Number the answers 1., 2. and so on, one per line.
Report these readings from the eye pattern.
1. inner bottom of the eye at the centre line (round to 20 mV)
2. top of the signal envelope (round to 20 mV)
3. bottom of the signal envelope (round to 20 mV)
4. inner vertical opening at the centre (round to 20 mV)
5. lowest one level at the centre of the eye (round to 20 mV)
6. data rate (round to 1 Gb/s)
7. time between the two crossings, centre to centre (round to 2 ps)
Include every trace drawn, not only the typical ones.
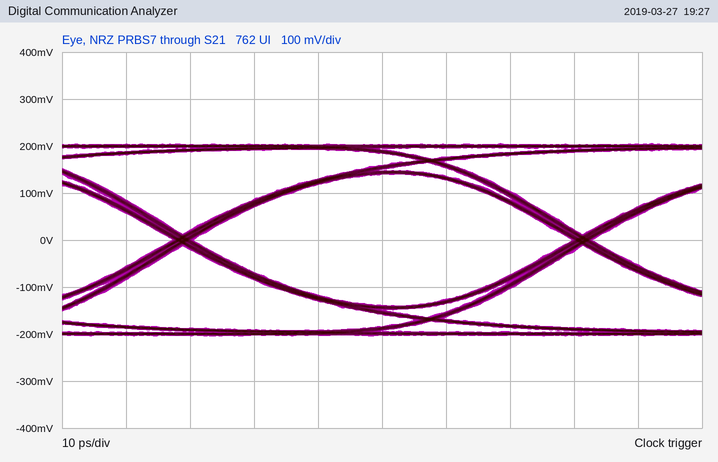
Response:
1. -140 mV
2. 200 mV
3. -200 mV
4. 280 mV
5. 140 mV
6. 16 Gb/s
7. 62 ps
